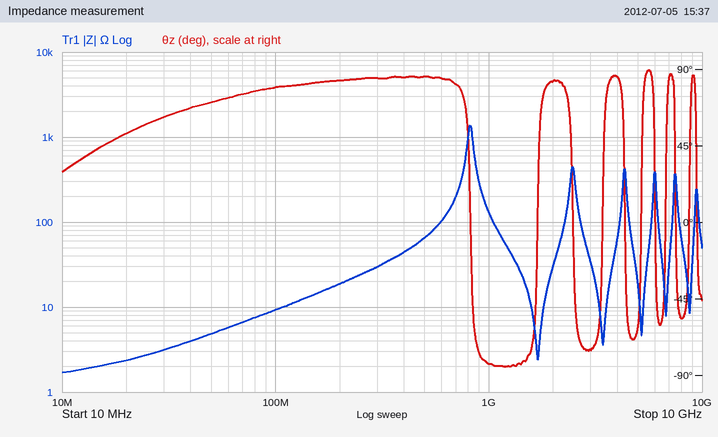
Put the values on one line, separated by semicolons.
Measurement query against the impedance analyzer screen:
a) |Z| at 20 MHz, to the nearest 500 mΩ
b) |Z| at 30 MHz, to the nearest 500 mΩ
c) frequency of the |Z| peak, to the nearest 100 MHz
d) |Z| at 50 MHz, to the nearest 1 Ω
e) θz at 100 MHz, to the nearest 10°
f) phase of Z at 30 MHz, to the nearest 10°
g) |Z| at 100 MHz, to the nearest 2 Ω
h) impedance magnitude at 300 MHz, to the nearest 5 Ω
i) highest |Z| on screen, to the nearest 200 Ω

2.5 Ω; 3.0 Ω; 800 MHz; 5 Ω; 80°; 60°; 10 Ω; 30 Ω; 1.4 kΩ
